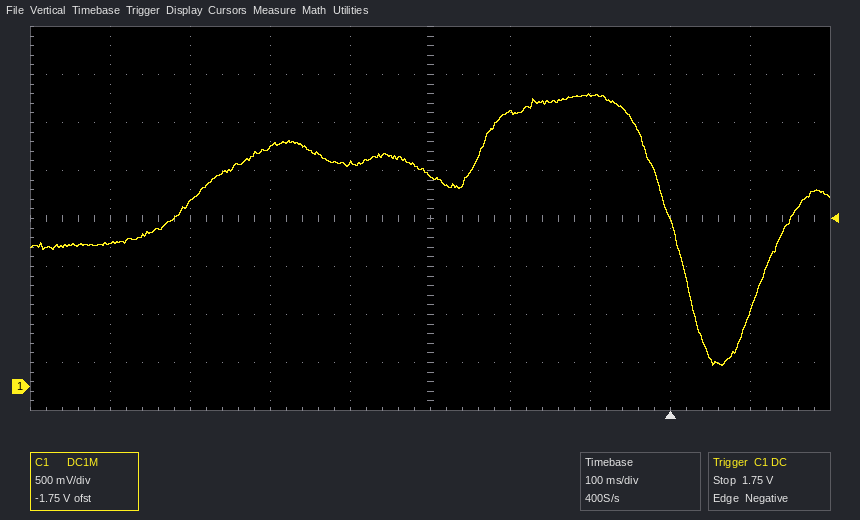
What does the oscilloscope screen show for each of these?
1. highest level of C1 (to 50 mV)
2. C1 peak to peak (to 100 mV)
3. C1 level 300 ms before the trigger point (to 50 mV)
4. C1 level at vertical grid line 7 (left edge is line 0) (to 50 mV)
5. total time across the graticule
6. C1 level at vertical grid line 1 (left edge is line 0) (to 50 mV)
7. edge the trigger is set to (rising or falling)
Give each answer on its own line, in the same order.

3.05 V
2.80 V
2.20 V
3.05 V
1 s
1.50 V
falling
